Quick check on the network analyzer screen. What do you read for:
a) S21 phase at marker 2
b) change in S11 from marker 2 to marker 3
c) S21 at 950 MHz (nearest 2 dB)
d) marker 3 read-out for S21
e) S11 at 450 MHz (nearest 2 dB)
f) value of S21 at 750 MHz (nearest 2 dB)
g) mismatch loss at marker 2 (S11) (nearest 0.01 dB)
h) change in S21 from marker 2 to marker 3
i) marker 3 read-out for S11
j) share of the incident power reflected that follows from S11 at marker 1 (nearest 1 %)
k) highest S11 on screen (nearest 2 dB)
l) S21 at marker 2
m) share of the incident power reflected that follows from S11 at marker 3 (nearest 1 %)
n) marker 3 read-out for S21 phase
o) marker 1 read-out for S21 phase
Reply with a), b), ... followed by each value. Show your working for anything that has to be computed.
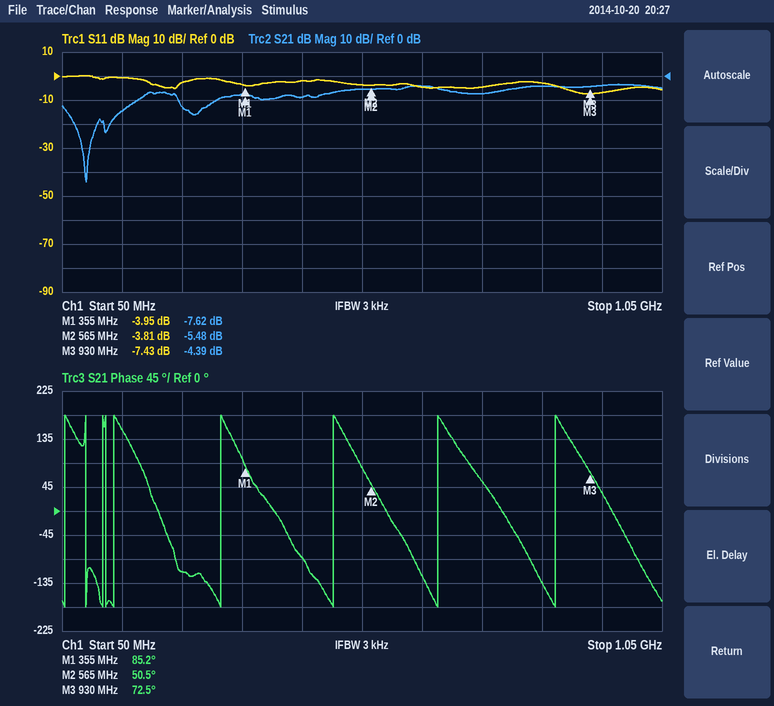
a) 50.5°
b) -7.43 − (-3.81) = -3.62 dB
c) -4 dB
d) -4.39 dB
e) -2 dB
f) -8 dB
g) −10 log10(1 − 10^(-3.81/10)) ≈ 2.34 dB
h) -4.39 − (-5.48) = 1.09 dB
i) -7.43 dB
j) 10^(-3.95/10) ≈ 40 %
k) 0 dB
l) -5.48 dB
m) 10^(-7.43/10) ≈ 18 %
n) 72.5°
o) 85.2°
